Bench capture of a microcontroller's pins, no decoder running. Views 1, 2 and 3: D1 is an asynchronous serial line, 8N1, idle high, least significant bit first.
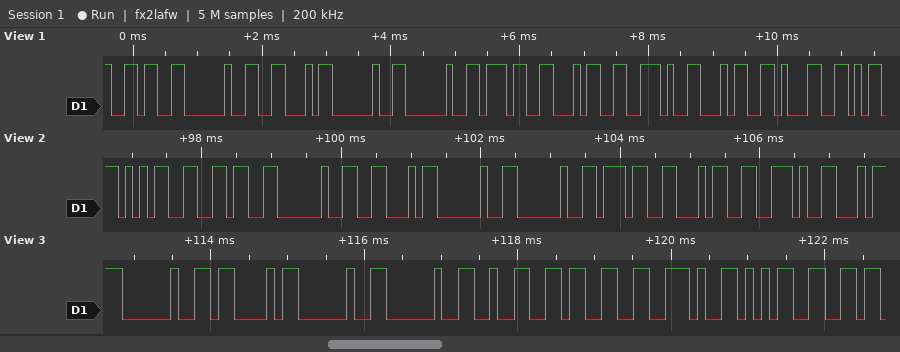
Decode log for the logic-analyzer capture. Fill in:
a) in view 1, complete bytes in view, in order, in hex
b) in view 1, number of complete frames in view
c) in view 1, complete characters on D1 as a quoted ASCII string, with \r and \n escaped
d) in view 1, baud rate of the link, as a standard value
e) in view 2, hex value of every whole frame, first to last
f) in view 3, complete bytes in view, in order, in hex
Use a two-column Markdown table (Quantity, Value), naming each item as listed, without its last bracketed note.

| Quantity | Value |
|---|---|
| in view 1, complete bytes in view, in order, in hex | 36 20 46 20 20 37 34 2E 34 31 |
| in view 1, number of complete frames in view | 10 |
| in view 1, complete characters on D1 as a quoted ASCII string, with \r and \n escaped | "6 F  74.41" |
| in view 1, baud rate of the link, as a standard value | 9600 baud |
| in view 2, hex value of every whole frame, first to last | 35 36 20 46 20 20 37 34 2E |
| in view 3, complete bytes in view, in order, in hex | 20 43 20 20 32 33 2E 35 |
